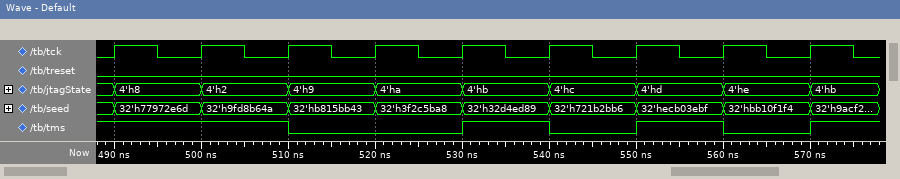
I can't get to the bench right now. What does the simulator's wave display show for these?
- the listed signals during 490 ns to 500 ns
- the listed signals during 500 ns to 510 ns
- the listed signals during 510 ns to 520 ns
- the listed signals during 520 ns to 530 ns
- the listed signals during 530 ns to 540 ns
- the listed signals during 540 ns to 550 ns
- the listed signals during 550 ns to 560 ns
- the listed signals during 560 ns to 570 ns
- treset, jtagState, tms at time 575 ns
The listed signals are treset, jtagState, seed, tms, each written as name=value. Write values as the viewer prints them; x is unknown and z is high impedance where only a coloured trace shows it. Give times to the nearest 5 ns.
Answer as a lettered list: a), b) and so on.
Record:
a) treset=0, jtagState=4'h8, seed=32'h77972e6d, tms=1
b) treset=0, jtagState=4'h2, seed=32'h9fd8b64a, tms=1
c) treset=0, jtagState=4'h9, seed=32'hb815bb43, tms=0
d) treset=0, jtagState=4'ha, seed=32'h3f2c5ba8, tms=0
e) treset=0, jtagState=4'hb, seed=32'h32d4ed89, tms=1
f) treset=0, jtagState=4'hc, seed=32'h721b2bb6, tms=0
g) treset=0, jtagState=4'hd, seed=32'hecb03ebf, tms=1
h) treset=0, jtagState=4'he, seed=32'hbb10f1f4, tms=0
i) treset=0, jtagState=4'hb, tms=1
